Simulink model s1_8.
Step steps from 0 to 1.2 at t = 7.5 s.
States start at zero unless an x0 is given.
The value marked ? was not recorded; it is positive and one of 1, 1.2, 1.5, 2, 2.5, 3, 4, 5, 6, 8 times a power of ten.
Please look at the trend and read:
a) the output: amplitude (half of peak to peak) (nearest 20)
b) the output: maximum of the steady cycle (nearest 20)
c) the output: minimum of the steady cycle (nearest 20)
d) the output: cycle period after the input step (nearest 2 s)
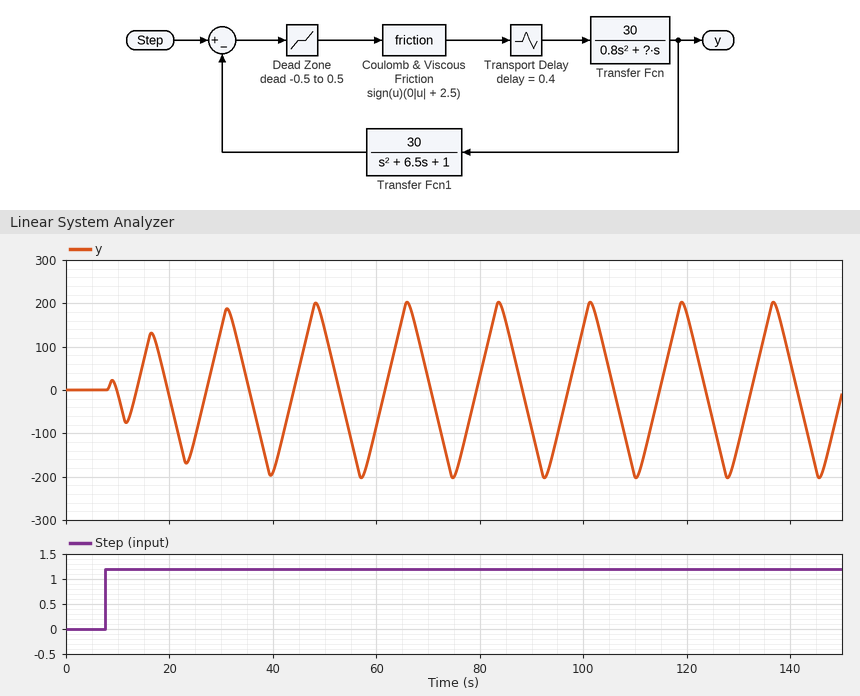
200
200
-200
18 s
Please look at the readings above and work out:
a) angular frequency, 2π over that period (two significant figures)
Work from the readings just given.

0.35 rad/s
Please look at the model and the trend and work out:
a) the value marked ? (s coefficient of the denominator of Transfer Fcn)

1.5
